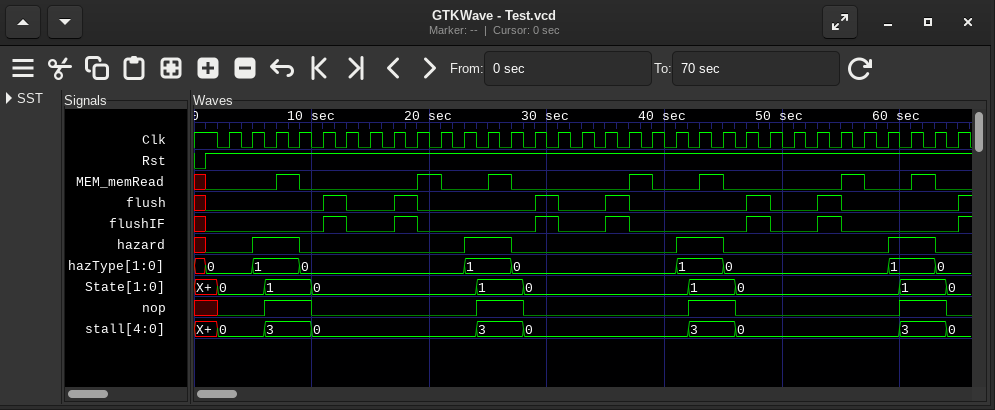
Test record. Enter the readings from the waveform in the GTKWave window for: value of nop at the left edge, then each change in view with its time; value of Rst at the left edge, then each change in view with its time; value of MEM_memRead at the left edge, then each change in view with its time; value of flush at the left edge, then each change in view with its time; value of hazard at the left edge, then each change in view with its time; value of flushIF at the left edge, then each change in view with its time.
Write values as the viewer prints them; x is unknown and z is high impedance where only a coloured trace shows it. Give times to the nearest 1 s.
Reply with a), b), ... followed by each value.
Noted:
a) x, 0 at 2 s, 1 at 6 s, 0 at 10 s, 1 at 24 s, 0 at 28 s, 1 at 42 s, 0 at 46 s, 1 at 60 s, 0 at 64 s
b) 0, 1 at 1 s
c) x, 0 at 1 s, 1 at 7 s, 0 at 9 s, 1 at 19 s, 0 at 21 s, 1 at 25 s, 0 at 27 s, 1 at 37 s, 0 at 39 s, 1 at 43 s, 0 at 45 s, 1 at 55 s, 0 at 57 s, 1 at 61 s, 0 at 63 s
d) x, 0 at 1 s, 1 at 11 s, 0 at 13 s, 1 at 17 s, 0 at 19 s, 1 at 29 s, 0 at 31 s, 1 at 35 s, 0 at 37 s, 1 at 47 s, 0 at 49 s, 1 at 53 s, 0 at 55 s, 1 at 65 s
e) x, 0 at 1 s, 1 at 5 s, 0 at 9 s, 1 at 23 s, 0 at 27 s, 1 at 41 s, 0 at 45 s, 1 at 59 s, 0 at 63 s
f) x, 0 at 1 s, 1 at 11 s, 0 at 13 s, 1 at 17 s, 0 at 19 s, 1 at 29 s, 0 at 31 s, 1 at 35 s, 0 at 37 s, 1 at 47 s, 0 at 49 s, 1 at 53 s, 0 at 55 s, 1 at 65 s
